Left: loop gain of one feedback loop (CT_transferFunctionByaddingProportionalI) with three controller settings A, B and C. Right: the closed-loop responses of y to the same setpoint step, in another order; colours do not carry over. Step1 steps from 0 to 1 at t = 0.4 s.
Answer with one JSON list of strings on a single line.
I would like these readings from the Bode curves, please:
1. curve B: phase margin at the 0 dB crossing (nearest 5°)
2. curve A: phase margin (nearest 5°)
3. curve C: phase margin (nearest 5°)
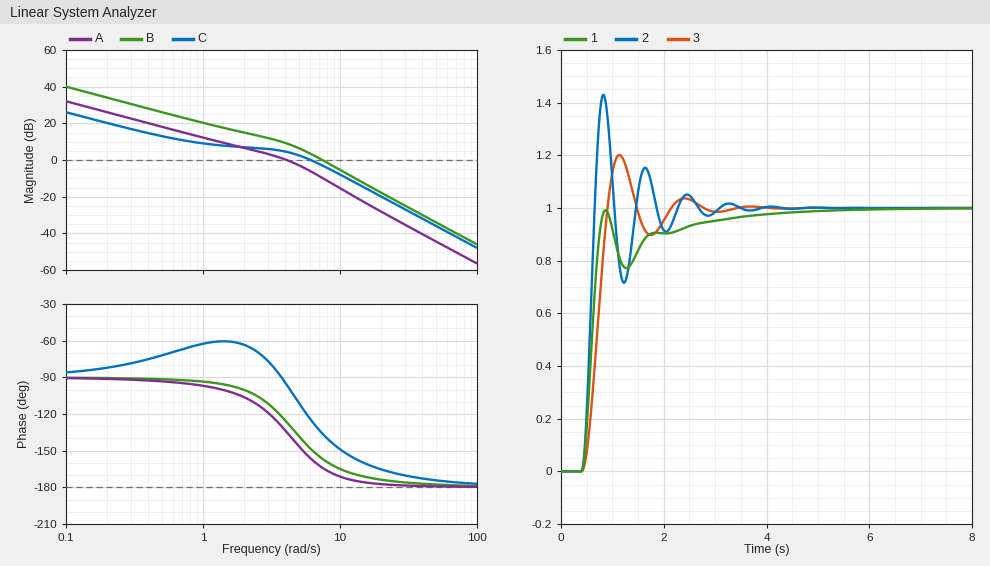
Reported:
["25°", "45°", "55°"]
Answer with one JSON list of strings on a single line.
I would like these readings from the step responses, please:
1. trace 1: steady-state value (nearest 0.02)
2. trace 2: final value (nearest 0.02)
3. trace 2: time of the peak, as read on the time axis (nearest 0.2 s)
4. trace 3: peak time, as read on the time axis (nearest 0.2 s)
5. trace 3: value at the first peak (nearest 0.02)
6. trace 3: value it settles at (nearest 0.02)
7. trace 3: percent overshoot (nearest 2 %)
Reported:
["1.00", "1.00", "0.8 s", "1.2 s", "1.20", "1.00", "20 %"]
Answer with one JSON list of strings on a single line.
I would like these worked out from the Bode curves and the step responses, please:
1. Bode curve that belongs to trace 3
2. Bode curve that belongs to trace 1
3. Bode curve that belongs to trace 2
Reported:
["A", "C", "B"]
